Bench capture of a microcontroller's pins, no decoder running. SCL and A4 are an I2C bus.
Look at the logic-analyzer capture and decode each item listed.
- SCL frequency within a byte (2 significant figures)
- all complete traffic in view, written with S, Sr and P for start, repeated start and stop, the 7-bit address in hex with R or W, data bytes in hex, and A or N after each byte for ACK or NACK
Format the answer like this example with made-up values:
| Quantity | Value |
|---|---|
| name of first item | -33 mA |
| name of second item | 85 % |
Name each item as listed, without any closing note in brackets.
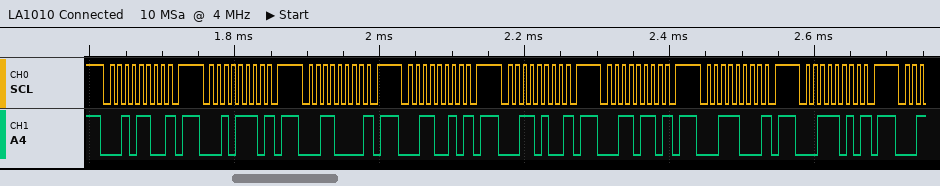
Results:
| Quantity | Value |
|---|---|
| SCL frequency within a byte | 100 kHz |
| all complete traffic in view, written with S, Sr and P for start, repeated start and stop, the 7-bit address in hex with R or W, data bytes in hex, and A or N after each byte for ACK or NACK | S 16W N P S 17W N P S 18W N P S 19W N P S 1AW N P S 1BW N P S 1CW N P S 1DW N P |
